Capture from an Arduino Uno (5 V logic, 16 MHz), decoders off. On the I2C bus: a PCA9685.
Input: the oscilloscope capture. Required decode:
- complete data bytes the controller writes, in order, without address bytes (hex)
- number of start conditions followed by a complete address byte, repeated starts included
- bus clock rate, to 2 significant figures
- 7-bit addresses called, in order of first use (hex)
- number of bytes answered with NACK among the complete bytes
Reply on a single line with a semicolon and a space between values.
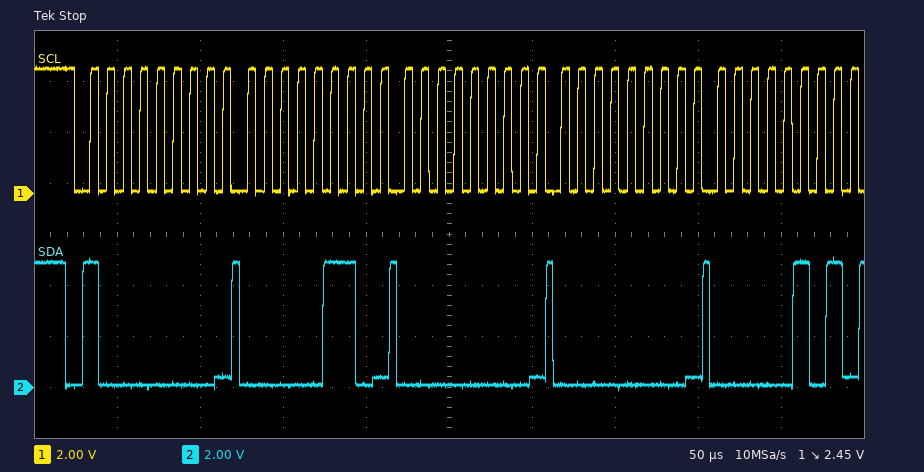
06 00 00 05; 1; 100 kHz; 0x40; 0
